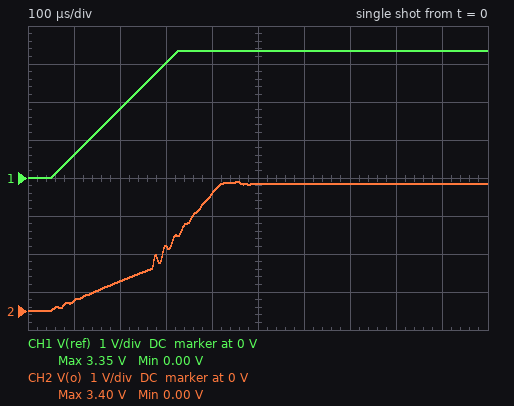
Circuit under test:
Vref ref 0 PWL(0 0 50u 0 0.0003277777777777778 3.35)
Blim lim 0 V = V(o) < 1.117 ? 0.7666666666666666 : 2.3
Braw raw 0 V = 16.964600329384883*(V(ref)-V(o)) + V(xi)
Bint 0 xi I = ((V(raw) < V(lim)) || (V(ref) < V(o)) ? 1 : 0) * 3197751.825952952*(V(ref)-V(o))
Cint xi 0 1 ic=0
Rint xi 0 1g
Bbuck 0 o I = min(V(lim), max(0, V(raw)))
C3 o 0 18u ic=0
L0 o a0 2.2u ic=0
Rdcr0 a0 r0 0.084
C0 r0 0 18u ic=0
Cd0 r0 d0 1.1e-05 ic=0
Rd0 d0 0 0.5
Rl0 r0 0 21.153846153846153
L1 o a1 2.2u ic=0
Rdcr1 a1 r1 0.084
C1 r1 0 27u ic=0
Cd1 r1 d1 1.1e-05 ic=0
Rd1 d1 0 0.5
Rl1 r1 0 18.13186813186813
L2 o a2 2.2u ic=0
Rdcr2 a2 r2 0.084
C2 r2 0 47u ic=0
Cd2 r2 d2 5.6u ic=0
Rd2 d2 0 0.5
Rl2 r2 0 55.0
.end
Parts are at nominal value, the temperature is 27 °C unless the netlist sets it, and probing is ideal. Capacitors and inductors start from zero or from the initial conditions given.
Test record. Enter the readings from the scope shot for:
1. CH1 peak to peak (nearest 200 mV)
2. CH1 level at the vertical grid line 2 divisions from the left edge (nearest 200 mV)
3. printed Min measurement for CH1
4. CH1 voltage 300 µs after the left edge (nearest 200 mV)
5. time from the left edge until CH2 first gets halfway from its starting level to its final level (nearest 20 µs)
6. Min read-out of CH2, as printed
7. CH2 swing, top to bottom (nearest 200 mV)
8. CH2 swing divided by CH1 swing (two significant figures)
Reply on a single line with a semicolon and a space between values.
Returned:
3.4 V; 1.8 V; 0.00 V; 3.0 V; 300 µs; 0.00 V; 3.4 V; 1.0
